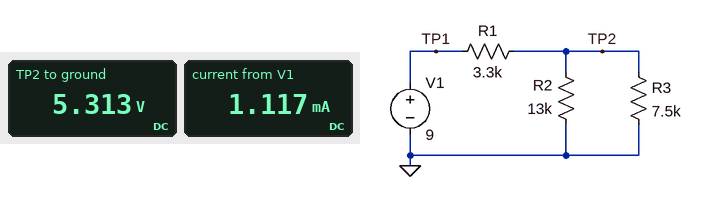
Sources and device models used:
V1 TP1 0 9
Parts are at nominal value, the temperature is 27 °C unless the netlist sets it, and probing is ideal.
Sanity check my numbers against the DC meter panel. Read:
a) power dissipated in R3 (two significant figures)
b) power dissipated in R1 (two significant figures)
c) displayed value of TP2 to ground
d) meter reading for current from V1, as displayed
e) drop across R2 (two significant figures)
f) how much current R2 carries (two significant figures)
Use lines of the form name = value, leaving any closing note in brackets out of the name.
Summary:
power dissipated in R3 = 3.8 mW
power dissipated in R1 = 4.1 mW
displayed value of TP2 to ground = 5.313 V
meter reading for current from V1, as displayed = 1.117 mA
drop across R2 = 5.3 V
how much current R2 carries = 410 µA
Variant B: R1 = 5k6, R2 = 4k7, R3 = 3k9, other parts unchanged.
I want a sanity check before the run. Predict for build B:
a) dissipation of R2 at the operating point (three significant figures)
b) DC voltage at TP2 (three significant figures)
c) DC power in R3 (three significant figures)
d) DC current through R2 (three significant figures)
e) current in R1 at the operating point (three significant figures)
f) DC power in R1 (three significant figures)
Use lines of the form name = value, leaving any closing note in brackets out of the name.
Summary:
dissipation of R2 at the operating point = 1.31 mW
DC voltage at TP2 = 2.48 V
DC power in R3 = 1.58 mW
DC current through R2 = 528 µA
current in R1 at the operating point = 1.16 mA
DC power in R1 = 7.59 mW
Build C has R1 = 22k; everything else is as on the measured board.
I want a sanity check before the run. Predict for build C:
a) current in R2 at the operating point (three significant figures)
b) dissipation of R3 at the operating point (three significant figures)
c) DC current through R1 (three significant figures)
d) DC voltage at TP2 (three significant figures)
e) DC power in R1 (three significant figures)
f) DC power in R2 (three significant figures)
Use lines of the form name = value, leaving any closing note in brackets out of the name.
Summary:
current in R2 at the operating point = 123 µA
dissipation of R3 at the operating point = 341 µW
DC current through R1 = 336 µA
DC voltage at TP2 = 1.60 V
DC power in R1 = 2.49 mW
DC power in R2 = 197 µW
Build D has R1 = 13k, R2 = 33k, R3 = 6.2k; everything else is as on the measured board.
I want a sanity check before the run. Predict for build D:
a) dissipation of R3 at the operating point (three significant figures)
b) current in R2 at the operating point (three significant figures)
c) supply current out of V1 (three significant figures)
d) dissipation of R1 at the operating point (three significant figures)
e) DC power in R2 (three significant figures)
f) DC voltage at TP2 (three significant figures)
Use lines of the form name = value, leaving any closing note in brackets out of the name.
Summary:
dissipation of R3 at the operating point = 1.07 mW
current in R2 at the operating point = 78.1 µA
supply current out of V1 = 494 µA
dissipation of R1 at the operating point = 3.17 mW
DC power in R2 = 201 µW
DC voltage at TP2 = 2.58 V
